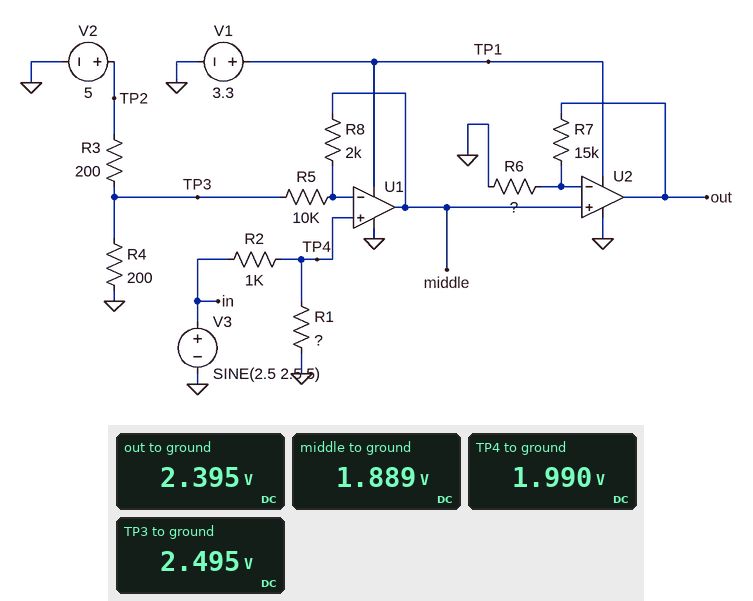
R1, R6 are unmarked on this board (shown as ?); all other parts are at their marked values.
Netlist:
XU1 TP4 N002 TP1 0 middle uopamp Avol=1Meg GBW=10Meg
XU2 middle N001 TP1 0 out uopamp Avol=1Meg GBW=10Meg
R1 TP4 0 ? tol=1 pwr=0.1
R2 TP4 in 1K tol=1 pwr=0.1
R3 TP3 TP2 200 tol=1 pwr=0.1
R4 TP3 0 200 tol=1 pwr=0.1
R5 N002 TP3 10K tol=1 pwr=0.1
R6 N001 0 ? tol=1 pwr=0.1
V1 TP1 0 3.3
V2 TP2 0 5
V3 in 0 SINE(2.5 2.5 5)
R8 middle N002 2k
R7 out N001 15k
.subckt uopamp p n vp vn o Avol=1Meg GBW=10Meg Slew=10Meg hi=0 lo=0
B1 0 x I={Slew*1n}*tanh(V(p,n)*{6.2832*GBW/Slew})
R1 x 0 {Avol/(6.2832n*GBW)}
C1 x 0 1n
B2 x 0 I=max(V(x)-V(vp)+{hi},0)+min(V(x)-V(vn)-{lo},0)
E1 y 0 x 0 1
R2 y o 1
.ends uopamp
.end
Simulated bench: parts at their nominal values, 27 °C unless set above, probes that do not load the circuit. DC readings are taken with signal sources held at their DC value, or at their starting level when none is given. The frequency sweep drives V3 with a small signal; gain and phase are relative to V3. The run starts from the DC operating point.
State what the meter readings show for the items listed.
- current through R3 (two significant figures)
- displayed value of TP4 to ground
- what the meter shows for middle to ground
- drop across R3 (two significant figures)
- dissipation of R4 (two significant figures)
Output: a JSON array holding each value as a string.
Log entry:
["13 mA", "1.990 V", "1.889 V", "2.5 V", "31 mW"]
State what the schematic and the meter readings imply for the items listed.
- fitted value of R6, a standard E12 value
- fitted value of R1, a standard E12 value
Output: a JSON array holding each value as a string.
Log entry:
["56 kΩ", "3.9 kΩ"]
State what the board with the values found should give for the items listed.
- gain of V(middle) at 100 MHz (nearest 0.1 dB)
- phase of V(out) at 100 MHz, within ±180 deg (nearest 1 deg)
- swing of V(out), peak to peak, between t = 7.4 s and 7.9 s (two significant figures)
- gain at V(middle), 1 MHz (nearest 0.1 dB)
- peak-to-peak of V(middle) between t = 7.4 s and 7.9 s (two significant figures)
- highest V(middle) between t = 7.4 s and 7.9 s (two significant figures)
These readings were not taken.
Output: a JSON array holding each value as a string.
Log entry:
["-22.0 dB", "-171 deg", "3.3 V", "-0.5 dB", "3.3 V", "3.3 V"]
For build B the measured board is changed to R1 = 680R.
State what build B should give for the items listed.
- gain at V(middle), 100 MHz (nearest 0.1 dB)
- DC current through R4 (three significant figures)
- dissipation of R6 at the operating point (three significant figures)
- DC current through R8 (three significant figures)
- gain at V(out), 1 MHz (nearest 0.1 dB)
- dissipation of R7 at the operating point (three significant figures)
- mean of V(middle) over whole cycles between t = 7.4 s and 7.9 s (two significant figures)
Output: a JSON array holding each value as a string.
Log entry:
["-27.9 dB", "12.4 mA", "9.19 µW", "147 µA", "-4.4 dB", "2.46 µW", "810 mV"]
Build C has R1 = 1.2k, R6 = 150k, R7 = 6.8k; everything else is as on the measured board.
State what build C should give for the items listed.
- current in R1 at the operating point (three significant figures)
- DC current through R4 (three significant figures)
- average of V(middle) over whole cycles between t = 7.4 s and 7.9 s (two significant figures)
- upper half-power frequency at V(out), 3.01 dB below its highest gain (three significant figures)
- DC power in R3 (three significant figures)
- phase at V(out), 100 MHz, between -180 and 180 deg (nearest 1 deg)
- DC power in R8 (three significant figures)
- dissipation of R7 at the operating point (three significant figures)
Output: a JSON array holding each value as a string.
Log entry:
["1.14 mA", "12.4 mA", "1.2 V", "5.73 MHz", "31.5 mW", "-170 deg", "25.3 µW", "392 nW"]
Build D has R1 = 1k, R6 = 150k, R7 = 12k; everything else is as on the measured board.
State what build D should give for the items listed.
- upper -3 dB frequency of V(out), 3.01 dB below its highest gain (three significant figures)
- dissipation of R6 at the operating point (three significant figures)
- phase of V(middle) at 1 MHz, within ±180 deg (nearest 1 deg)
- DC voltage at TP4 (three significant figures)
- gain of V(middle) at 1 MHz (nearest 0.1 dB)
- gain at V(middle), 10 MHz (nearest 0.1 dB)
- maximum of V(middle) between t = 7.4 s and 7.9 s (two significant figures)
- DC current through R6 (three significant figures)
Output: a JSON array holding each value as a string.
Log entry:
["5.65 MHz", "6.70 µW", "-7 deg", "1.25 V", "-4.5 dB", "-8.3 dB", "2.5 V", "6.68 µA"]
